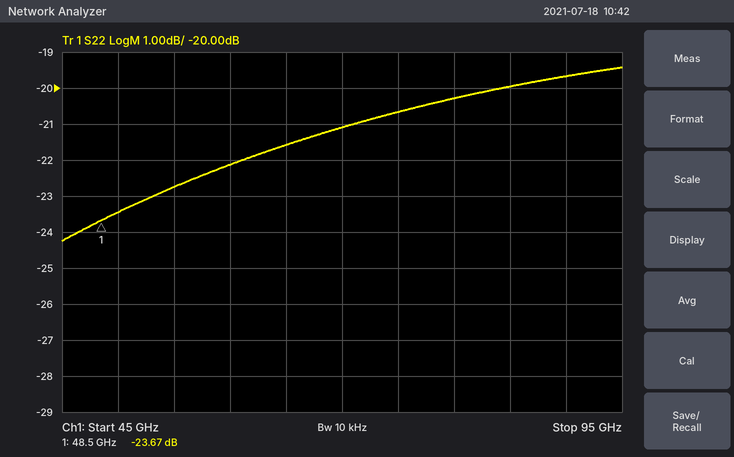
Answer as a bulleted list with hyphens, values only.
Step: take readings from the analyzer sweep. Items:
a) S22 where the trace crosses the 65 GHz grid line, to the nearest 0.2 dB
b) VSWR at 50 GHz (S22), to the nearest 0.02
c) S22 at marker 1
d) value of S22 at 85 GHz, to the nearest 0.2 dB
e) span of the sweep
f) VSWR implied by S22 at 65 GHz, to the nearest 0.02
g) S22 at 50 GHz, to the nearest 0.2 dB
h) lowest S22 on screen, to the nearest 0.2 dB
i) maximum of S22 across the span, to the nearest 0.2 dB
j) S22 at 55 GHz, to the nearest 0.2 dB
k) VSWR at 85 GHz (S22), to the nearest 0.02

- -21.6 dB
- 1.14
- -23.67 dB
- -20.0 dB
- 50 GHz
- 1.18
- -23.4 dB
- -24.2 dB
- -19.4 dB
- -22.8 dB
- 1.22
